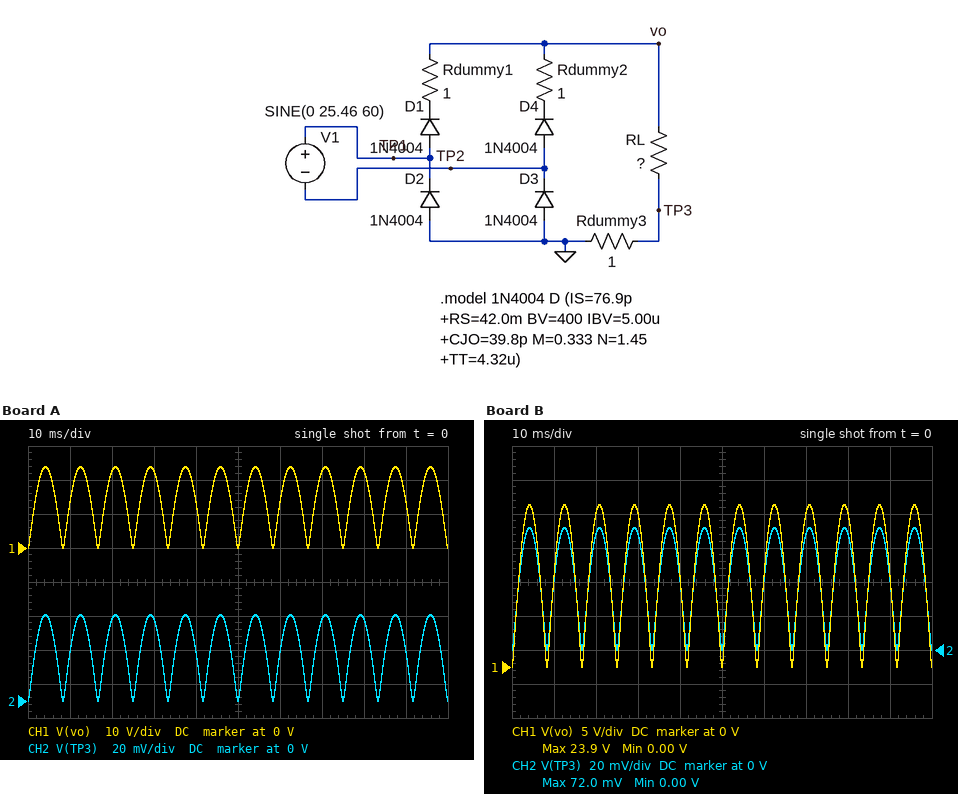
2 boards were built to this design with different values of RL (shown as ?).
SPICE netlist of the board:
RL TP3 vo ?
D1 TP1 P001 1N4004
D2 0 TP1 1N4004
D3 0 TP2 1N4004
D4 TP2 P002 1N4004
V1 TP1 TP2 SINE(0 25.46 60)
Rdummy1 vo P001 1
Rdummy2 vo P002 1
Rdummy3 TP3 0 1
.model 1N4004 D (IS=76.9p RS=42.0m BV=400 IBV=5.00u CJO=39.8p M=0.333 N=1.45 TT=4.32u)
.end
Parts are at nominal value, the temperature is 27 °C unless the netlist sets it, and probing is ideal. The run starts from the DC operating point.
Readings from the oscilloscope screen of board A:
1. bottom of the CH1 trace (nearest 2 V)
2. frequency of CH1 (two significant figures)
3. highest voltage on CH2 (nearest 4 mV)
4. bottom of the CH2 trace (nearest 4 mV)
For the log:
0 V
120 Hz
52 mV
0 V
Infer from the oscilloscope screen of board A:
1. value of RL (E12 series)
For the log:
470 Ω
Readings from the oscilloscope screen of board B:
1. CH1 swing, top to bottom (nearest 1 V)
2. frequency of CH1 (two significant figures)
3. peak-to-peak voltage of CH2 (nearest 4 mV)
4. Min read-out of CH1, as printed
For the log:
24 V
120 Hz
72 mV
0.00 V
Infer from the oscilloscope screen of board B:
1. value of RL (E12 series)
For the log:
330 Ω
